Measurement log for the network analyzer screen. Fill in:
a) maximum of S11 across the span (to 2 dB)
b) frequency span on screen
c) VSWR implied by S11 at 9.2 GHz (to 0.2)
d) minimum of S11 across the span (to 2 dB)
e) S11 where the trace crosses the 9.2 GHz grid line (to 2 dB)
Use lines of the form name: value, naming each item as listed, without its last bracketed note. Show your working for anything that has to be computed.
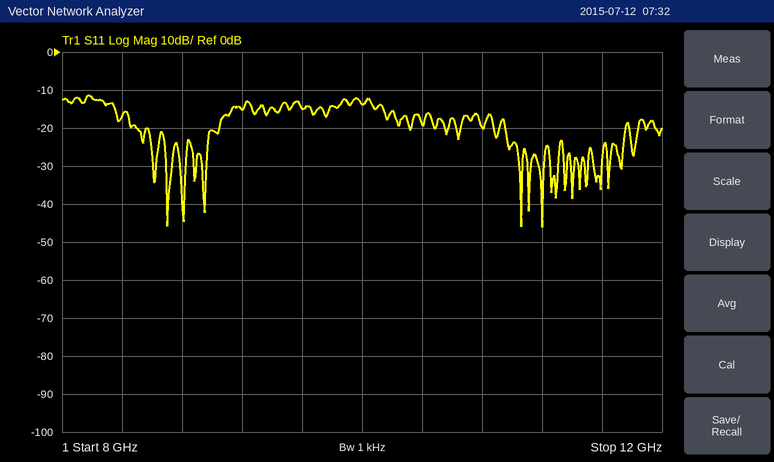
maximum of S11 across the span: -12 dB
frequency span on screen: 4 GHz
VSWR implied by S11 at 9.2 GHz: |Γ| = 10^(-16/20) = 0.1585; VSWR = (1 + 0.1585)/(1 − 0.1585) ≈ 1.4
minimum of S11 across the span: -46 dB
S11 where the trace crosses the 9.2 GHz grid line: -16 dB
